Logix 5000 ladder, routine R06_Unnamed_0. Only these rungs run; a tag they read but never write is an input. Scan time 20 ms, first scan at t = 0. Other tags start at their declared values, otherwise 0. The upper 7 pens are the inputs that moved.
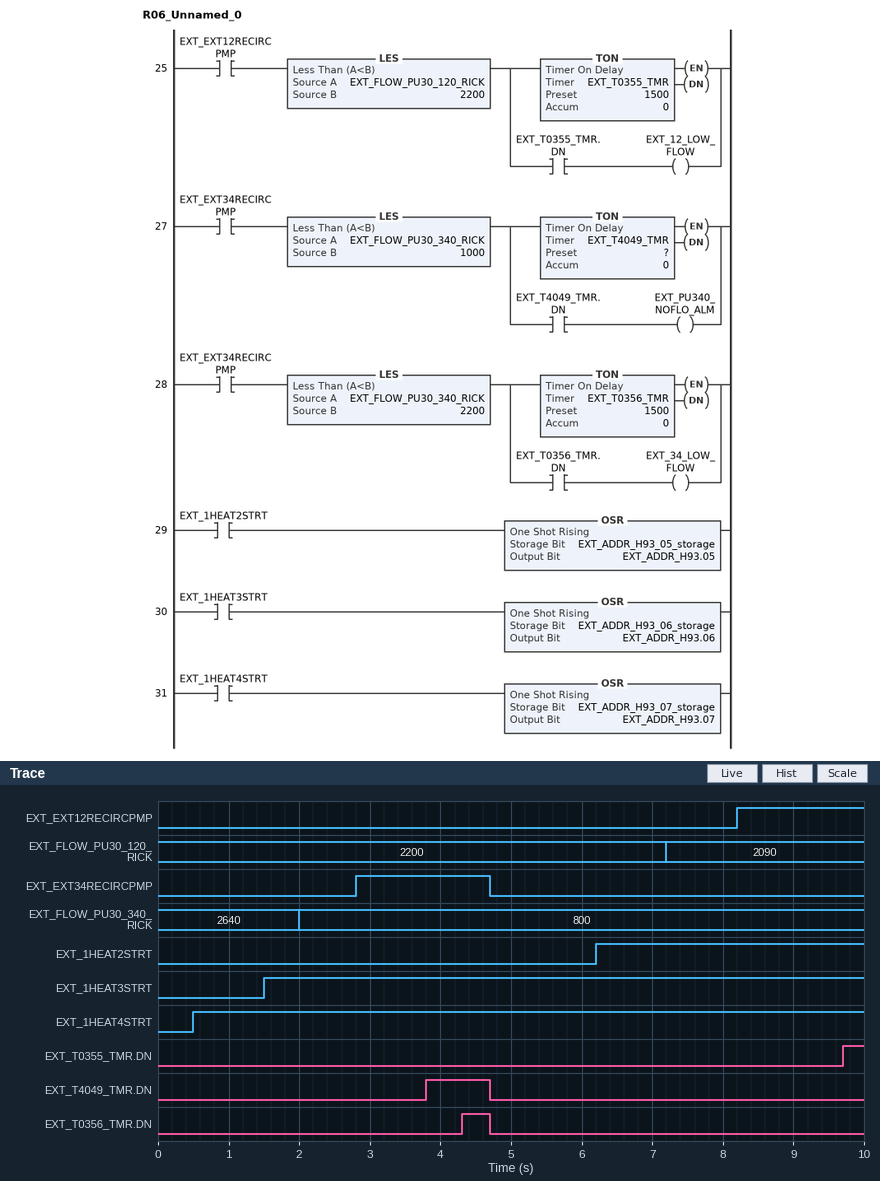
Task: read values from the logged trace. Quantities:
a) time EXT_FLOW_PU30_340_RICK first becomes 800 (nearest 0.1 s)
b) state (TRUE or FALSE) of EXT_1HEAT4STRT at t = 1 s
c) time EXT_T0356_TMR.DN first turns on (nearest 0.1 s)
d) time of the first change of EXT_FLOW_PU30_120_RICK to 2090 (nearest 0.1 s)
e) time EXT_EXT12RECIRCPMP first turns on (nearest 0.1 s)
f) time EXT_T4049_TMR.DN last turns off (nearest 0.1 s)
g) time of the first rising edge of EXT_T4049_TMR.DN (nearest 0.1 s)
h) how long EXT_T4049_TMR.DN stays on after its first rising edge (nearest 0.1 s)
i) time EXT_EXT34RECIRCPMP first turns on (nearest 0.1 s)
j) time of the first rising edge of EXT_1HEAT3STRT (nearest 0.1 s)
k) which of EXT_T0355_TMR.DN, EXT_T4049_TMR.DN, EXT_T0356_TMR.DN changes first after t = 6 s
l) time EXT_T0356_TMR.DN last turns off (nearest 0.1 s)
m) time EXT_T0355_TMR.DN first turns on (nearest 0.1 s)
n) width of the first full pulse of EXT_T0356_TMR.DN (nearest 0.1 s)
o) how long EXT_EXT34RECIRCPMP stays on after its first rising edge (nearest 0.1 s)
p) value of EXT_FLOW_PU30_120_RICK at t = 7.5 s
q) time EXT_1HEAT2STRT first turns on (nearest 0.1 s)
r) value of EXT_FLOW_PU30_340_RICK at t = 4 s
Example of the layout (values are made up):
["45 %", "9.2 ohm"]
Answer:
["2.0 s", "TRUE", "4.3 s", "7.2 s", "8.2 s", "4.7 s", "3.8 s", "0.9 s", "2.8 s", "1.5 s", "EXT_T0355_TMR.DN", "4.7 s", "9.7 s", "0.4 s", "1.9 s", "2090", "6.2 s", "800"]
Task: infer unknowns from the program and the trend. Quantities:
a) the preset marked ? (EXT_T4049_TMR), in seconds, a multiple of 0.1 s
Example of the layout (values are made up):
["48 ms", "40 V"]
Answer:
["1.0 s"]
